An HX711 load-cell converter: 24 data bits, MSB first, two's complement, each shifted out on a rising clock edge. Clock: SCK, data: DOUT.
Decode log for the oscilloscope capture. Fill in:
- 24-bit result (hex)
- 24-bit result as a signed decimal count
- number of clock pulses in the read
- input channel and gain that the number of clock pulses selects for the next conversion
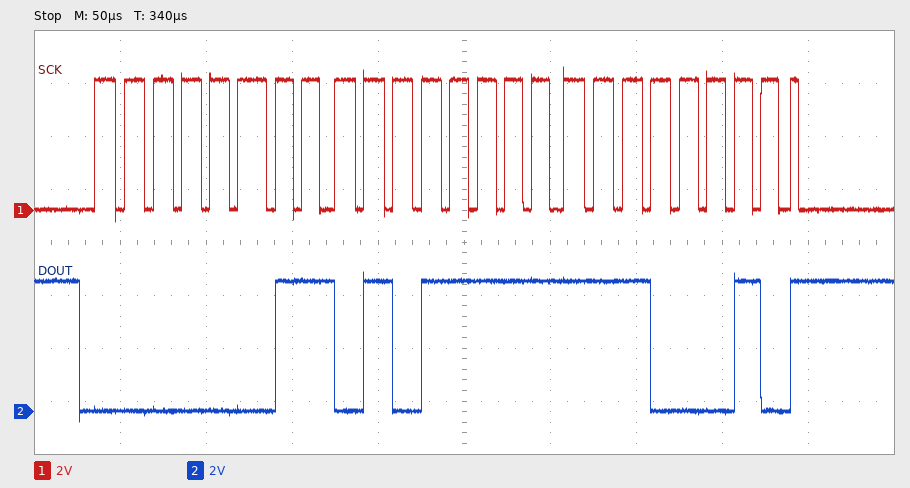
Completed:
0x035FE2
221154
25
channel A, gain 128
